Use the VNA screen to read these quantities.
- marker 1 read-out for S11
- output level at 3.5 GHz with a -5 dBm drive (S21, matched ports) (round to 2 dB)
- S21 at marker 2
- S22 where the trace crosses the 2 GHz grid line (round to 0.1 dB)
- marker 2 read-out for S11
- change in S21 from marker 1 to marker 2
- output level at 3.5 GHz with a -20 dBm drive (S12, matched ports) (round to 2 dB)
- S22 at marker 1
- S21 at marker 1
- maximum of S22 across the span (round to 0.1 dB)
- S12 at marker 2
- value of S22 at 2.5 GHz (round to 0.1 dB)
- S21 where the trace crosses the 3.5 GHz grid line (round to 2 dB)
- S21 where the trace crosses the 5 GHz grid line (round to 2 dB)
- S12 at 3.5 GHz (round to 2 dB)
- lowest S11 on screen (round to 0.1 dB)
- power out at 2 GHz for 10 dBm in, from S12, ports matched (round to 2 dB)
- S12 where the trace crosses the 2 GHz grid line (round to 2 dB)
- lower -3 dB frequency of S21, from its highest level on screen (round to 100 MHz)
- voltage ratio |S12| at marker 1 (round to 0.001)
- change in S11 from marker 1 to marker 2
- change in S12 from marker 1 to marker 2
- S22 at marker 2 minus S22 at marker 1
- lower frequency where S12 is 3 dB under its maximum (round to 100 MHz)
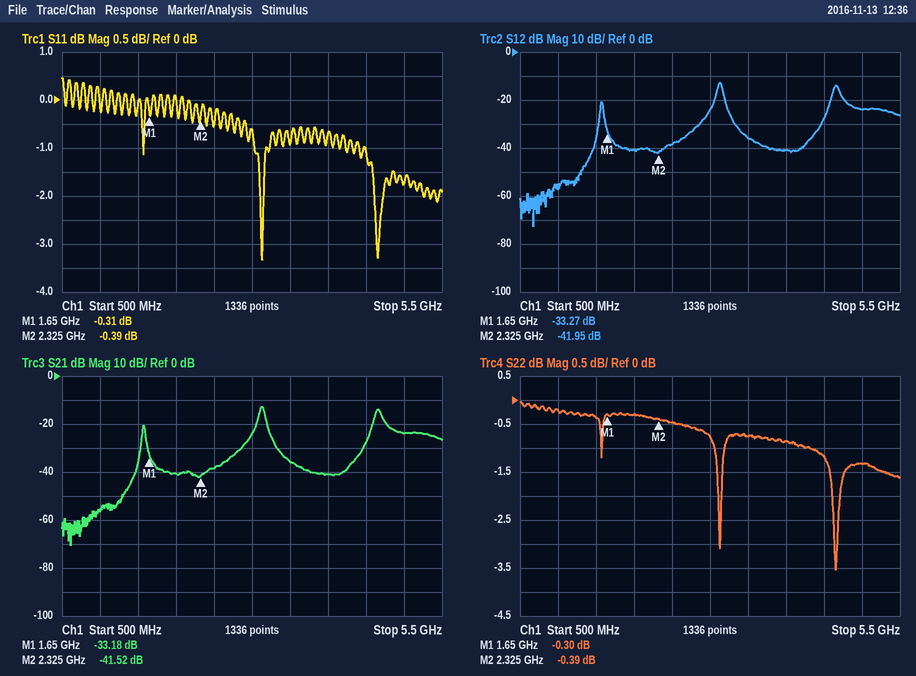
-0.31 dB
-40 dBm
-41.52 dB
-0.3 dB
-0.39 dB
-8.34 dB
-56 dBm
-0.30 dB
-33.18 dB
0.0 dB
-41.95 dB
-0.5 dB
-36 dB
-24 dB
-36 dB
-3.3 dB
-30 dBm
-40 dB
3.1 GHz
0.022
-0.08 dB
-8.68 dB
-0.09 dB
3.1 GHz
